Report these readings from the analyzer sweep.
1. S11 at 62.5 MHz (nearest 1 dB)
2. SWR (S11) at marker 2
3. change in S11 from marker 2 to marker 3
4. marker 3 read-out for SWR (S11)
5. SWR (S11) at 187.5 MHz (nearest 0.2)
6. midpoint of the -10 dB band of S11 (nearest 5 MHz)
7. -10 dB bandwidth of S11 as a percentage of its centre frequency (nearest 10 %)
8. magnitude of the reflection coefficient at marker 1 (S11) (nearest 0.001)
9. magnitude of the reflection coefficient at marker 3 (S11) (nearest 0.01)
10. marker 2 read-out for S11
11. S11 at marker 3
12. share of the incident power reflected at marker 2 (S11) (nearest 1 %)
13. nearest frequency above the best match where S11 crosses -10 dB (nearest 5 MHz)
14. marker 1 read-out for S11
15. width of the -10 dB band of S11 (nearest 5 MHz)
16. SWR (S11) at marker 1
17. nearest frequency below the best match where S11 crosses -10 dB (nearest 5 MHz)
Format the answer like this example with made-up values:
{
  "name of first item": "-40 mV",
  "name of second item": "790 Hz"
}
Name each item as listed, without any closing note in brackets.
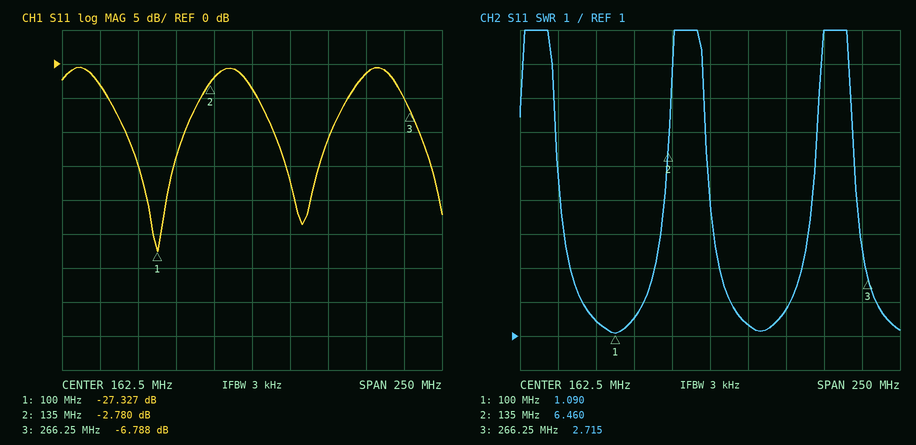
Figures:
{
  "S11 at 62.5 MHz": "-3 dB",
  "SWR (S11) at marker 2": "6.460",
  "change in S11 from marker 2 to marker 3": "-4.008 dB",
  "marker 3 read-out for SWR": "2.715",
  "SWR (S11) at 187.5 MHz": "1.4",
  "midpoint of the -10 dB band of S11": "100 MHz",
  "-10 dB bandwidth of S11 as a percentage of its centre frequency": "40 %",
  "magnitude of the reflection coefficient at marker 1 (S11)": "0.043",
  "magnitude of the reflection coefficient at marker 3 (S11)": "0.46",
  "marker 2 read-out for S11": "-2.780 dB",
  "S11 at marker 3": "-6.788 dB",
  "share of the incident power reflected at marker 2 (S11)": "53 %",
  "nearest frequency above the best match where S11 crosses -10 dB": "120 MHz",
  "marker 1 read-out for S11": "-27.327 dB",
  "width of the -10 dB band of S11": "40 MHz",
  "SWR (S11) at marker 1": "1.090",
  "nearest frequency below the best match where S11 crosses -10 dB": "80 MHz"
}
